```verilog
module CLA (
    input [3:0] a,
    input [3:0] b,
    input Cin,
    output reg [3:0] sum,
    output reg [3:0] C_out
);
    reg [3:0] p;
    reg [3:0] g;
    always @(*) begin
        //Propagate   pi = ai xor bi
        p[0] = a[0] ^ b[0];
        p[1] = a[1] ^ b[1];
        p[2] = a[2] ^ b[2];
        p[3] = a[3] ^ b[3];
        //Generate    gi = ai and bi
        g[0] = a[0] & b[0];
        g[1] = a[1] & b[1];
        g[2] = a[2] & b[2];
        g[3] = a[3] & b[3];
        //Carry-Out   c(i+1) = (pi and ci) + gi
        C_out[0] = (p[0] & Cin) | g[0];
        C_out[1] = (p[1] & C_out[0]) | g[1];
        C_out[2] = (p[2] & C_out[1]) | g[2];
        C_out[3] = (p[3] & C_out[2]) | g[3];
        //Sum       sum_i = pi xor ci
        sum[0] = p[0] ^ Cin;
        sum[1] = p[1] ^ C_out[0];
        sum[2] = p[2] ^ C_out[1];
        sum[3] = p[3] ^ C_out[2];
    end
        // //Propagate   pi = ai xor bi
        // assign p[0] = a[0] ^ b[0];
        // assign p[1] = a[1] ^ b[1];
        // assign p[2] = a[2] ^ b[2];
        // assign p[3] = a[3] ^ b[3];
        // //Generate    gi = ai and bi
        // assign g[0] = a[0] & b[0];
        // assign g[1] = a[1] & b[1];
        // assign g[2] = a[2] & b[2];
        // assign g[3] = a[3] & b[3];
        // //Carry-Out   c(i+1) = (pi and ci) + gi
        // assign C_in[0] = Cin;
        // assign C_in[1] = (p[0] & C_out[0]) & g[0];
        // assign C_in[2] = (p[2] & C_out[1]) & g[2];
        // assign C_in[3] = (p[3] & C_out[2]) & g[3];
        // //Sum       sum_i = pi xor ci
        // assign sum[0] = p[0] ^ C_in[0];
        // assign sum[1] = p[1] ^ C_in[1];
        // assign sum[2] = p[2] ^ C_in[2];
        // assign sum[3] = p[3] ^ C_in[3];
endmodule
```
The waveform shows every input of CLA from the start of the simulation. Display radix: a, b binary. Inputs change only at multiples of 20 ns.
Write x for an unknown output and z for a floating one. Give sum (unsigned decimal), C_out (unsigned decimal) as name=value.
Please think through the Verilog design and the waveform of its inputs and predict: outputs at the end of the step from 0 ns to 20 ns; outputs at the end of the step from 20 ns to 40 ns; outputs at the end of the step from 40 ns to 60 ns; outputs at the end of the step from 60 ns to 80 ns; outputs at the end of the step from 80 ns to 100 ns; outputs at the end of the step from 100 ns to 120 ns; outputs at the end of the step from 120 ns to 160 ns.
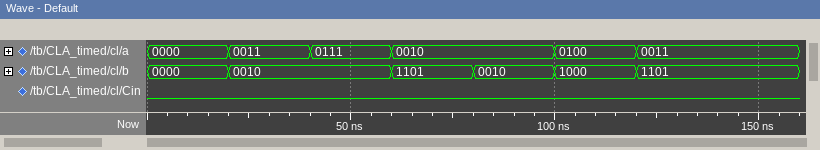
sum=0, C_out=0
sum=5, C_out=2
sum=9, C_out=6
sum=15, C_out=0
sum=4, C_out=2
sum=12, C_out=0
sum=0, C_out=15
